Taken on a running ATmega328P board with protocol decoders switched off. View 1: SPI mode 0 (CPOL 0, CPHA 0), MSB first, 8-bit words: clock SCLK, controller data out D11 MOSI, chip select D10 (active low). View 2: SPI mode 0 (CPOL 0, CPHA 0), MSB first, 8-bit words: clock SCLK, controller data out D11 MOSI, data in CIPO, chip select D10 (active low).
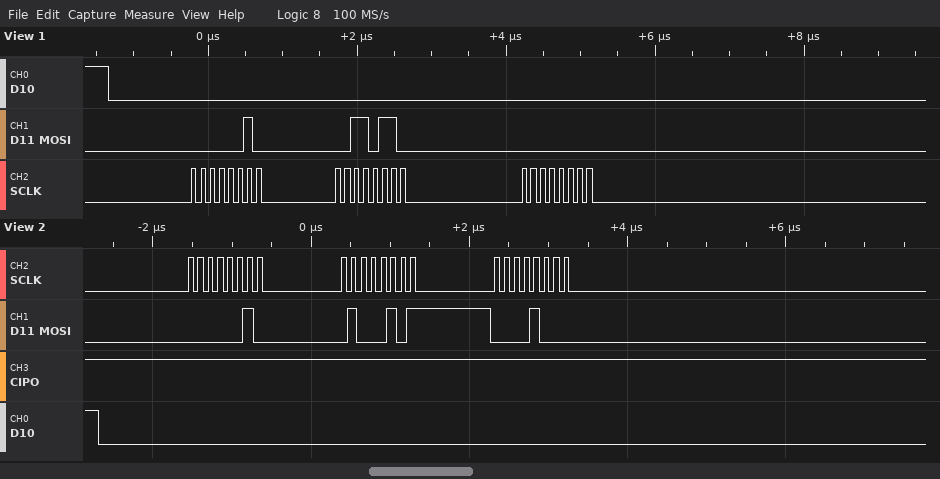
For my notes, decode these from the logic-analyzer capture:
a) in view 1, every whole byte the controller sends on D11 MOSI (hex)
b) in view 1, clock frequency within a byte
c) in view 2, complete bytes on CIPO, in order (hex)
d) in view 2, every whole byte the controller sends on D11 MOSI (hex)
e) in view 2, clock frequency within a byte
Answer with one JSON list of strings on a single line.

["02 36 00", "8 MHz", "0xFF 0xFF 0xFF", "0x02 0x45 0x08", "8 MHz"]
